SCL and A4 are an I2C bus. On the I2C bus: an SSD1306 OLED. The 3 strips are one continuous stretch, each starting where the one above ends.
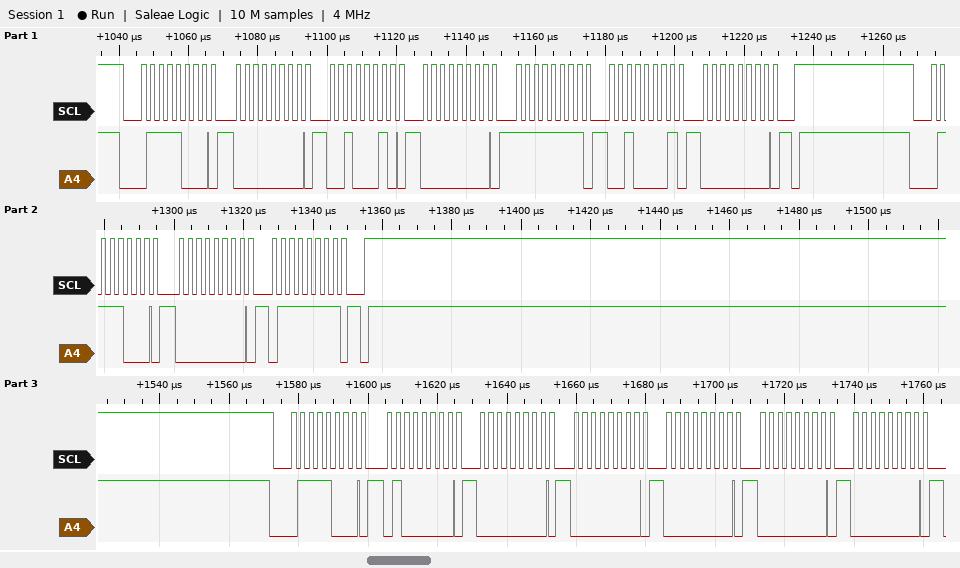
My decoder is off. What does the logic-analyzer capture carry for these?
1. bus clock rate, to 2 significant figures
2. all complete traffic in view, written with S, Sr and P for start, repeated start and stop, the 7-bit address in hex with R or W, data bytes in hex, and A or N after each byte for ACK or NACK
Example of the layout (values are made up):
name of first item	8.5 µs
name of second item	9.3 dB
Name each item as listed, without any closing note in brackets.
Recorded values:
bus clock rate, to 2 significant figures	400 kHz
all complete traffic in view, written with S, Sr and P for start, repeated start and stop, the 7-bit address in hex with R or W, data bytes in hex, and A or N after each byte for ACK or NACK	S 3CW A 00 A 22 A 00 A FF A 21 A 00 A P S 3CW A 00 A 7F A P S 3CW A 40 A 00 A 00 A 00 A 00 A 00 A
